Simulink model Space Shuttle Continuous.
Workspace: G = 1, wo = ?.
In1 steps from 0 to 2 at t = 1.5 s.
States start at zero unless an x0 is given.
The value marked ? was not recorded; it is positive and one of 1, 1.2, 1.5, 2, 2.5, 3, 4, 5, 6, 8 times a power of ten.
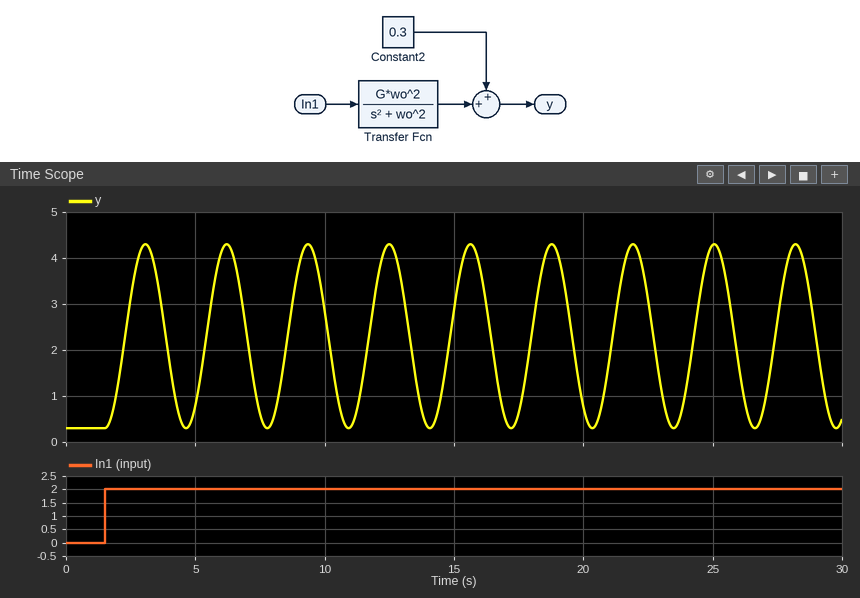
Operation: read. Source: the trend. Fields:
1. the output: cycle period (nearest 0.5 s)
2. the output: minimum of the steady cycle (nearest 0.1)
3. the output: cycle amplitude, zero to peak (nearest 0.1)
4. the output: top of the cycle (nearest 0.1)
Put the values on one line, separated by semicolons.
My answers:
3.0 s; 0.3; 2.0; 4.3
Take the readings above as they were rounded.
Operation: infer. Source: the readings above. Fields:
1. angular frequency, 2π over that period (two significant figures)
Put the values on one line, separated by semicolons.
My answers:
2.1 rad/s
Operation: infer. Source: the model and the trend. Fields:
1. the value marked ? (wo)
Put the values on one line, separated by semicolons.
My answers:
2
